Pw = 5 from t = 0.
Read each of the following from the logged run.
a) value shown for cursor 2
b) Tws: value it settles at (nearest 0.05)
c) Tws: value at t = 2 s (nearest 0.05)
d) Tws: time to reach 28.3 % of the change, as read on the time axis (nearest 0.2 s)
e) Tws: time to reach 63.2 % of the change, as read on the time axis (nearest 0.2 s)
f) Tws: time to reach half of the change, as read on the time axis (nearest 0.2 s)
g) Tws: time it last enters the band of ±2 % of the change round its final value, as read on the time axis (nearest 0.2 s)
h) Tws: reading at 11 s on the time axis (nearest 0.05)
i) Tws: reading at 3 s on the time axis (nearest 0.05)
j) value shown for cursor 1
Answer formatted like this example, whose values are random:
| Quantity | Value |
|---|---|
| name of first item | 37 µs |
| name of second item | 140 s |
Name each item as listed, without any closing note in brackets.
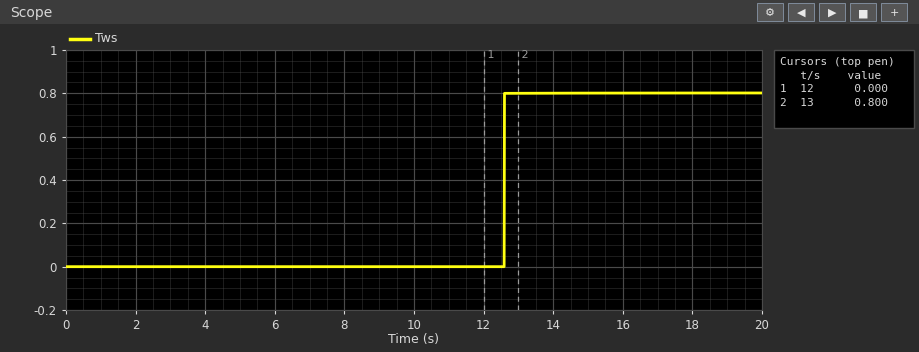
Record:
| Quantity | Value |
|---|---|
| value shown for cursor 2 | 0.800 |
| Tws: value it settles at | 0.80 |
| Tws: value at t = 2 s | 0.00 |
| Tws: time to reach 28.3 % of the change, as read on the time axis | 12.6 s |
| Tws: time to reach 63.2 % of the change, as read on the time axis | 12.6 s |
| Tws: time to reach half of the change, as read on the time axis | 12.6 s |
| Tws: time it last enters the band of ±2 % of the change round its final value, as read on the time axis | 12.6 s |
| Tws: reading at 11 s on the time axis | 0.00 |
| Tws: reading at 3 s on the time axis | 0.00 |
| value shown for cursor 1 | 0.000 |
